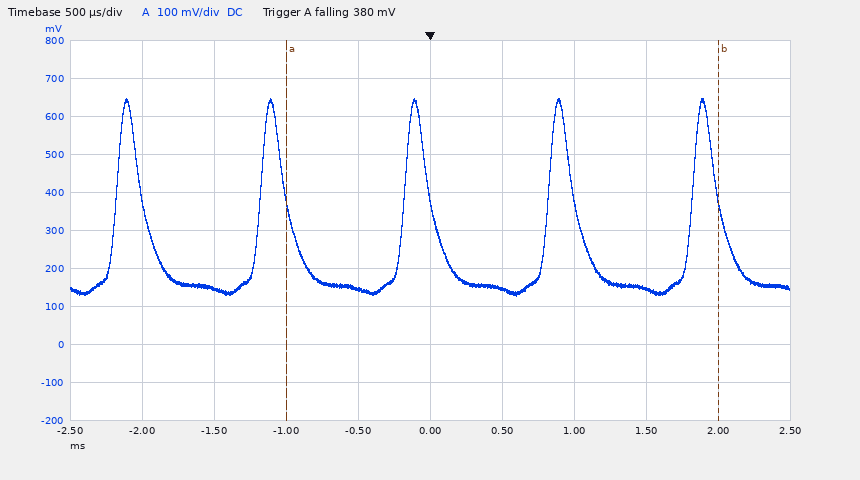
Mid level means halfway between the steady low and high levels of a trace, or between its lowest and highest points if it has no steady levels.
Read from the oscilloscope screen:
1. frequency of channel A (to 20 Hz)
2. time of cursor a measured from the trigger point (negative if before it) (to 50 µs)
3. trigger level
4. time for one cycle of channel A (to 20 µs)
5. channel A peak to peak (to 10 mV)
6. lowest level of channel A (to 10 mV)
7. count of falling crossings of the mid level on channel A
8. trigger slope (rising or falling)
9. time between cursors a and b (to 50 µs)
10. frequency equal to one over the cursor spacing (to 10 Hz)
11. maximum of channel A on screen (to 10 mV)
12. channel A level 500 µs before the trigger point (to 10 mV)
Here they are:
1.00 kHz
-1.00 ms
380 mV
1.00 ms
520 mV
130 mV
5
falling
3.00 ms
330 Hz
650 mV
150 mV
